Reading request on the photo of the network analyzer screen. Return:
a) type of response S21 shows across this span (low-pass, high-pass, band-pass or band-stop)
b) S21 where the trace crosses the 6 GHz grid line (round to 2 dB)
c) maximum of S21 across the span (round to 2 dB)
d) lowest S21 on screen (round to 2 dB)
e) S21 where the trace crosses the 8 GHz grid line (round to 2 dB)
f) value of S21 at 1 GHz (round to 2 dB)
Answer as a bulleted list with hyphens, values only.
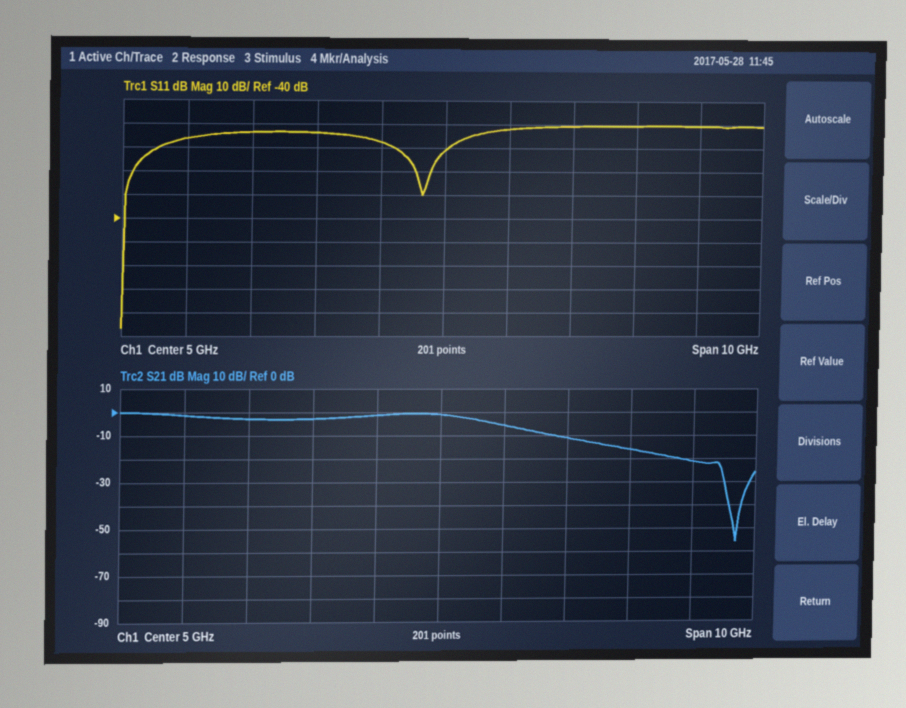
- low-pass
- -6 dB
- 0 dB
- -56 dB
- -16 dB
- -2 dB
